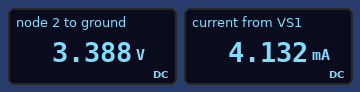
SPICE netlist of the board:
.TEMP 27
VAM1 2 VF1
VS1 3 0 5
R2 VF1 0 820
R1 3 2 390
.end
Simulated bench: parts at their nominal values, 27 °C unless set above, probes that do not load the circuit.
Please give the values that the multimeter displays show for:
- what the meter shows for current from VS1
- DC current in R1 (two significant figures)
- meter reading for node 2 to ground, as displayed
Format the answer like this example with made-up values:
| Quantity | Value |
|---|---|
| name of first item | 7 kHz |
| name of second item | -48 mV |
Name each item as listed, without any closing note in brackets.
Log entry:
| Quantity | Value |
|---|---|
| what the meter shows for current from VS1 | 4.132 mA |
| DC current in R1 | 4.1 mA |
| meter reading for node 2 to ground, as displayed | 3.388 V |
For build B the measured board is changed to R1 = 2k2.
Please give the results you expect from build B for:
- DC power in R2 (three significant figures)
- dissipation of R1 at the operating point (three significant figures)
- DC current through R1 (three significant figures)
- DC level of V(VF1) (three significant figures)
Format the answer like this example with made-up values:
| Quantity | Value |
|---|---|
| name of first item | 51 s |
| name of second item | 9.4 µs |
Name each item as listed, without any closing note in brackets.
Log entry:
| Quantity | Value |
|---|---|
| DC power in R2 | 2.25 mW |
| dissipation of R1 at the operating point | 6.03 mW |
| DC current through R1 | 1.66 mA |
| DC level of V(VF1) | 1.36 V |
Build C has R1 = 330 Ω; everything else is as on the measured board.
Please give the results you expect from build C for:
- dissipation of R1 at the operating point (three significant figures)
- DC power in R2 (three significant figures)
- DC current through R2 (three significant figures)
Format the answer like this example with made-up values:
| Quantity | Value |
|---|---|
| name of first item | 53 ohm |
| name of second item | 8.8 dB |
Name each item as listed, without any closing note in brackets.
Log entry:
| Quantity | Value |
|---|---|
| dissipation of R1 at the operating point | 6.24 mW |
| DC power in R2 | 15.5 mW |
| DC current through R2 | 4.35 mA |
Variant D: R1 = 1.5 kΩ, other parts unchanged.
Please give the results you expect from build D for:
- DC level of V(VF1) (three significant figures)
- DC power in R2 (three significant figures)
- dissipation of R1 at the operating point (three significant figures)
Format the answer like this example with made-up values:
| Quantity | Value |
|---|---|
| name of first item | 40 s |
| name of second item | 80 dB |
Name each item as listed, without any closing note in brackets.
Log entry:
| Quantity | Value |
|---|---|
| DC level of V(VF1) | 1.77 V |
| DC power in R2 | 3.81 mW |
| dissipation of R1 at the operating point | 6.97 mW |
